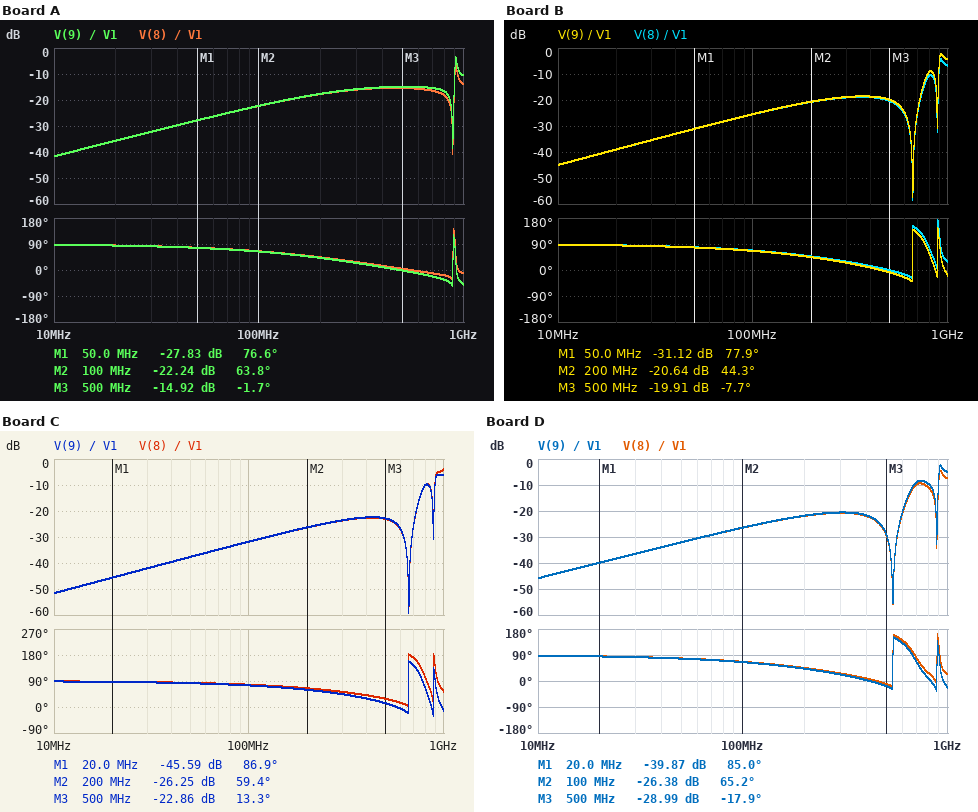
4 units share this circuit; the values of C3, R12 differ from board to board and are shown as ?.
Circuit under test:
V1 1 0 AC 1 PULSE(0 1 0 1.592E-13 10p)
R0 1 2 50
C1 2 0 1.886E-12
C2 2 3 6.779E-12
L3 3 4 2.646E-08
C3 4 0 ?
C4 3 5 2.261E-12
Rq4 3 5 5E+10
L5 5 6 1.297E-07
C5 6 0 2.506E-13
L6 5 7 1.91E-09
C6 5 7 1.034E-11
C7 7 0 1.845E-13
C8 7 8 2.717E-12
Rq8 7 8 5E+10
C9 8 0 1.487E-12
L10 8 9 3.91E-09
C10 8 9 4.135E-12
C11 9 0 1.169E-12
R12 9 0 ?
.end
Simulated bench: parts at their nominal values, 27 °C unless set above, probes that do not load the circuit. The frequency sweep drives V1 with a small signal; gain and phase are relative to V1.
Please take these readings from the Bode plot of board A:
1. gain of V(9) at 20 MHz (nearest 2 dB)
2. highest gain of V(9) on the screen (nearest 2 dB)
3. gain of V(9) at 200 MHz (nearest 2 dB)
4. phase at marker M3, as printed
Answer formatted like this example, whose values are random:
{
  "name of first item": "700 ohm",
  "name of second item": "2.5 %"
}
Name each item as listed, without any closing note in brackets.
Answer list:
{
  "gain of V(9) at 20 MHz": "-36 dB",
  "highest gain of V(9) on the screen": "-4 dB",
  "gain of V(9) at 200 MHz": "-18 dB",
  "phase at marker M3, as printed": "-1.7 deg"
}
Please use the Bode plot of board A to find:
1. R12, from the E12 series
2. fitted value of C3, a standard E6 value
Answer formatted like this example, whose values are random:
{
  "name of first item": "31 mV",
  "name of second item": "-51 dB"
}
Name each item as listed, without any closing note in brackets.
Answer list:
{
  "R12, from the E12 series": "150 Ω",
  "fitted value of C3, a standard E6 value": "680 fF"
}
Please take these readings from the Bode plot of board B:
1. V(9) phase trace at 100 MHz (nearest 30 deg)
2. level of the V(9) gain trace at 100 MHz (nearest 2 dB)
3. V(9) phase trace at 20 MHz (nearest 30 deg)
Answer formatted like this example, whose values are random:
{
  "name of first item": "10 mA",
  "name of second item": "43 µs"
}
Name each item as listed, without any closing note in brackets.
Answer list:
{
  "V(9) phase trace at 100 MHz": "60 deg",
  "level of the V(9) gain trace at 100 MHz": "-26 dB",
  "V(9) phase trace at 20 MHz": "90 deg"
}
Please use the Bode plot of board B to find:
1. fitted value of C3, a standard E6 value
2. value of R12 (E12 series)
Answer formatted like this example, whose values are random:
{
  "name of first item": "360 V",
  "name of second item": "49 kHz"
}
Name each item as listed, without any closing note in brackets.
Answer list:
{
  "fitted value of C3, a standard E6 value": "2.2 pF",
  "value of R12": "120 Ω"
}
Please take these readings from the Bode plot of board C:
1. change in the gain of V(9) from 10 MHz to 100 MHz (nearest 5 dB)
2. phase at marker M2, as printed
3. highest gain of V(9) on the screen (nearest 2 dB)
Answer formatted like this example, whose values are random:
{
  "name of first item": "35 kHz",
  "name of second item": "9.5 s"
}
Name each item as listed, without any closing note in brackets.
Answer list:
{
  "change in the gain of V(9) from 10 MHz to 100 MHz": "20 dB",
  "phase at marker M2, as printed": "59.4 deg",
  "highest gain of V(9) on the screen": "-6 dB"
}
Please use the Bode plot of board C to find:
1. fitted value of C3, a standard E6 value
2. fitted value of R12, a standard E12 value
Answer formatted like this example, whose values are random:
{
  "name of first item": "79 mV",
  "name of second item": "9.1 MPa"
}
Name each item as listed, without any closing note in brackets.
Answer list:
{
  "fitted value of C3, a standard E6 value": "2.2 pF",
  "fitted value of R12, a standard E12 value": "56 Ω"
}
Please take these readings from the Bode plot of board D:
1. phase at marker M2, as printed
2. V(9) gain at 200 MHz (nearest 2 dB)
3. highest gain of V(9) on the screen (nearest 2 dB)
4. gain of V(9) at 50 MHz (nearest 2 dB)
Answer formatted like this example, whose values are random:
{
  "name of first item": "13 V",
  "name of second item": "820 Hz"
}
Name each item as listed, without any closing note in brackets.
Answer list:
{
  "phase at marker M2, as printed": "65.2 deg",
  "V(9) gain at 200 MHz": "-22 dB",
  "highest gain of V(9) on the screen": "-2 dB",
  "gain of V(9) at 50 MHz": "-32 dB"
}
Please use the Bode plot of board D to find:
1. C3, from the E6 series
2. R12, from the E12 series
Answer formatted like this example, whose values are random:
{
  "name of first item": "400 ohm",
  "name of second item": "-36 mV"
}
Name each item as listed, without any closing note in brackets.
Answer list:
{
  "C3, from the E6 series": "3.3 pF",
  "R12, from the E12 series": "120 Ω"
}
